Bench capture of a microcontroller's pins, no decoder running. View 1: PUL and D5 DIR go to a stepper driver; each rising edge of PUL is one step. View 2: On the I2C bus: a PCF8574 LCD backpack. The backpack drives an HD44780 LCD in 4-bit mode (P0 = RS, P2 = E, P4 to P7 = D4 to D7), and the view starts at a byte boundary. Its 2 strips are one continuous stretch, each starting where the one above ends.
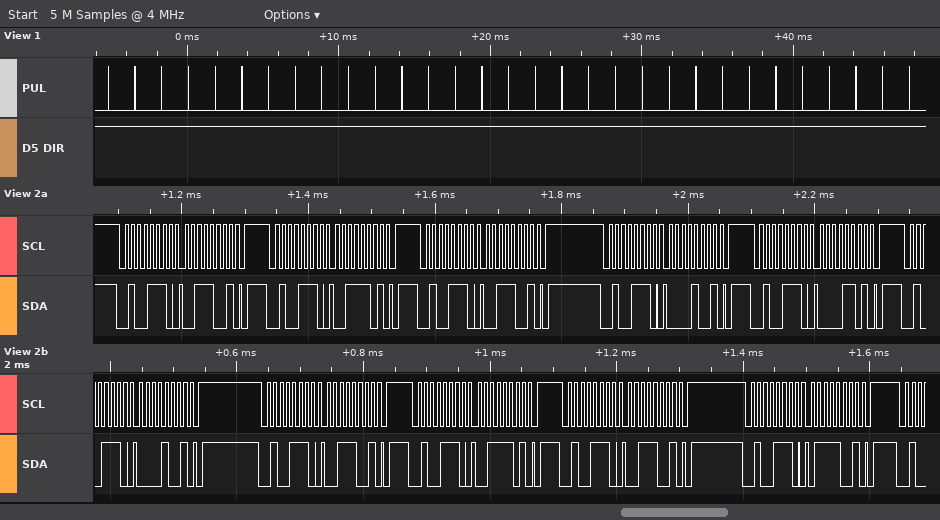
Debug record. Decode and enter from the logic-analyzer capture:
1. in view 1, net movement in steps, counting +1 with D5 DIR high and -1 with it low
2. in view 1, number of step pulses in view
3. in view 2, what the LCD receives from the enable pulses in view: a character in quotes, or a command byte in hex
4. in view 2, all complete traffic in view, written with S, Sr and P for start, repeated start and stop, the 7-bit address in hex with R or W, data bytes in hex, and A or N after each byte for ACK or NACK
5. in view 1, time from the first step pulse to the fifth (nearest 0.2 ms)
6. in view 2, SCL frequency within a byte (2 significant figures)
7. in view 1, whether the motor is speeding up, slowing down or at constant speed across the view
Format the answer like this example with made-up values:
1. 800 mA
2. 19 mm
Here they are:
1. +31
2. 31
3. '0'
4. S 27W A 39 A P S 27W A 3D A P S 27W A 39 A P S 27W A 09 A P S 27W A 0D A P S 27W A 09 A P S 27W A 39 A P S 27W A 3D A P S 27W A 39 A P S 27W A 79 A P
5. 7.0 ms
6. 100 kHz
7. constant speed
